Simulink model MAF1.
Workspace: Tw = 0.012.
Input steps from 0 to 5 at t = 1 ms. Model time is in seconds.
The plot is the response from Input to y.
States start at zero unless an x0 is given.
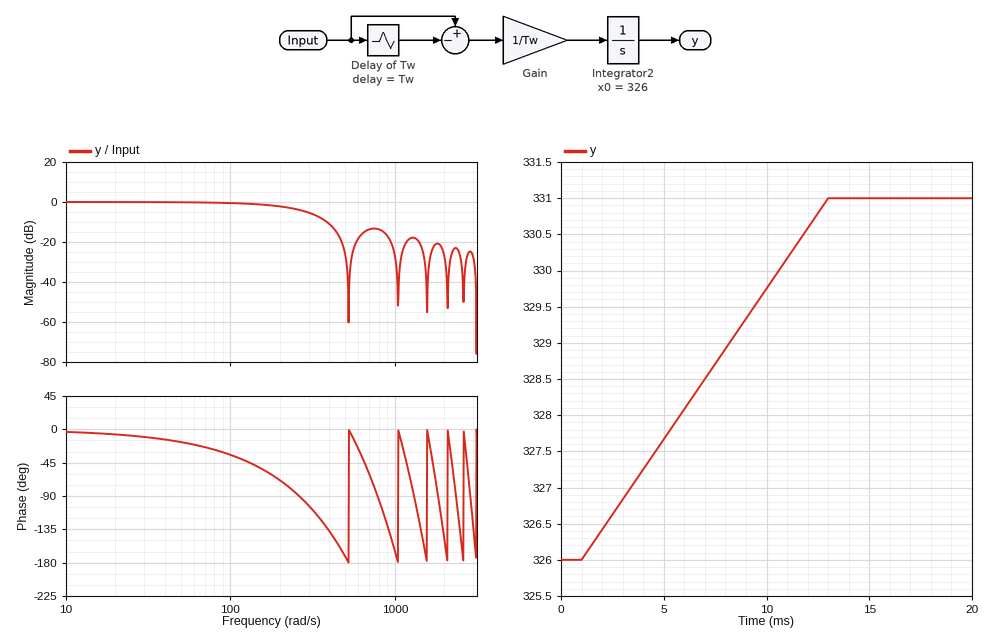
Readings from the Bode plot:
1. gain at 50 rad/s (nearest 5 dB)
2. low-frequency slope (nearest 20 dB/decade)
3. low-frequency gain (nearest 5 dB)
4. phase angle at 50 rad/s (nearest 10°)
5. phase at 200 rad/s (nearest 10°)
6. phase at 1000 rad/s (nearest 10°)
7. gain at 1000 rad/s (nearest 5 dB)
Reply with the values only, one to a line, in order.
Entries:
0 dB
0 dB/decade
0 dB
-20°
-70°
-160°
-25 dB
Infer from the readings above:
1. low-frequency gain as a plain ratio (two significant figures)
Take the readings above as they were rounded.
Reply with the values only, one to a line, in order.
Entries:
1.0
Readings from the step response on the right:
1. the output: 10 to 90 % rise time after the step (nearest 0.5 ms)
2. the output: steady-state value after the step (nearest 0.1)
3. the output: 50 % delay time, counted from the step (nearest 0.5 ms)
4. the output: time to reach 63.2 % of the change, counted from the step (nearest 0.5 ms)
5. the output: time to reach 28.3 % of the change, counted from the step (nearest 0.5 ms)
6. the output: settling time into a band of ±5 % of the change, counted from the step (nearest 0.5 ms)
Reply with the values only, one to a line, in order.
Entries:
9.5 ms
331.0
6.0 ms
7.5 ms
3.5 ms
11.5 ms
